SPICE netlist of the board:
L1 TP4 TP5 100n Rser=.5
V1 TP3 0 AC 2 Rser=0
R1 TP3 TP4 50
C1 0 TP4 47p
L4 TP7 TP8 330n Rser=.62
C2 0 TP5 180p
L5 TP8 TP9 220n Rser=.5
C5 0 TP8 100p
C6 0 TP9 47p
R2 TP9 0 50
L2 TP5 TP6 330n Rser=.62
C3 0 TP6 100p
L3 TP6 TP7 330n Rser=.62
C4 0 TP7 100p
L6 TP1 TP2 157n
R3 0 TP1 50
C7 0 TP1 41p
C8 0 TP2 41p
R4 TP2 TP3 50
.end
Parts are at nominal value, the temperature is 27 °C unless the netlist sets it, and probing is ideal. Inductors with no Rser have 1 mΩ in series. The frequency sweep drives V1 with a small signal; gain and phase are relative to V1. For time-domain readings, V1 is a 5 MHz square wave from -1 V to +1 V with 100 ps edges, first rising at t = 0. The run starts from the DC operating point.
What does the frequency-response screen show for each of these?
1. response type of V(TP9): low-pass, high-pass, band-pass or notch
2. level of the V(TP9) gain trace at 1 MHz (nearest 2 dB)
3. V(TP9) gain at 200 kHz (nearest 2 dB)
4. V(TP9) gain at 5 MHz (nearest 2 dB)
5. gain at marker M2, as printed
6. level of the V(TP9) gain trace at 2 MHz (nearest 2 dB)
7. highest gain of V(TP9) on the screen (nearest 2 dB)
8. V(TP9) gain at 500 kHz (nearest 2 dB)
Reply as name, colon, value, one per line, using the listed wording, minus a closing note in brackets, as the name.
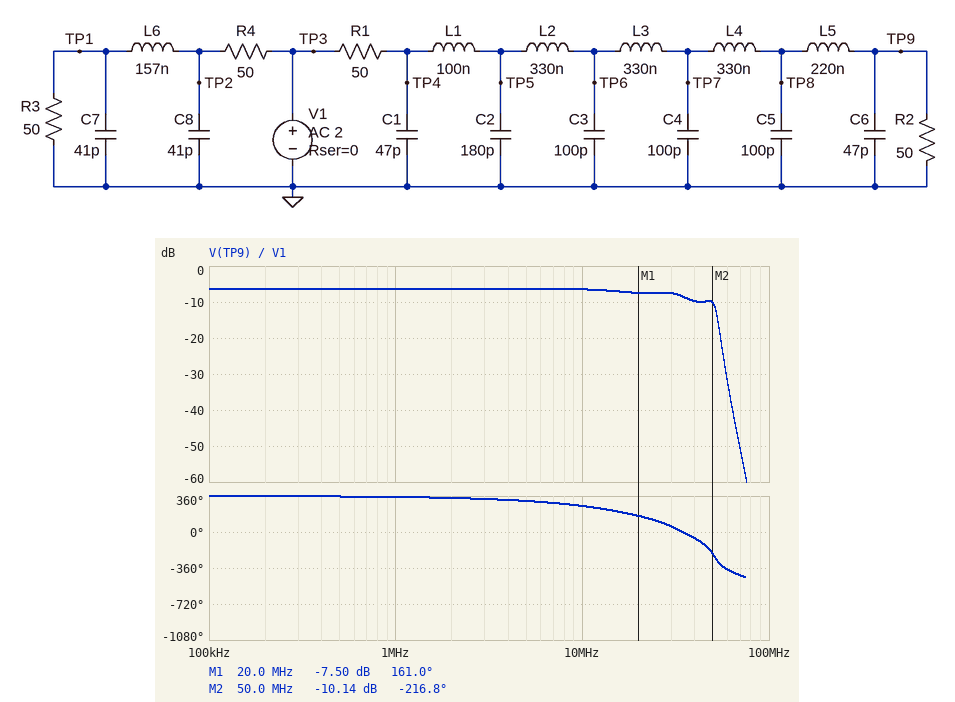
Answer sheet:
response type of V(TP9): low-pass, high-pass, band-pass or notch: low-pass
level of the V(TP9) gain trace at 1 MHz: -6 dB
V(TP9) gain at 200 kHz: -6 dB
V(TP9) gain at 5 MHz: -6 dB
gain at marker M2, as printed: -10.14 dB
level of the V(TP9) gain trace at 2 MHz: -6 dB
highest gain of V(TP9) on the screen: -6 dB
V(TP9) gain at 500 kHz: -6 dB
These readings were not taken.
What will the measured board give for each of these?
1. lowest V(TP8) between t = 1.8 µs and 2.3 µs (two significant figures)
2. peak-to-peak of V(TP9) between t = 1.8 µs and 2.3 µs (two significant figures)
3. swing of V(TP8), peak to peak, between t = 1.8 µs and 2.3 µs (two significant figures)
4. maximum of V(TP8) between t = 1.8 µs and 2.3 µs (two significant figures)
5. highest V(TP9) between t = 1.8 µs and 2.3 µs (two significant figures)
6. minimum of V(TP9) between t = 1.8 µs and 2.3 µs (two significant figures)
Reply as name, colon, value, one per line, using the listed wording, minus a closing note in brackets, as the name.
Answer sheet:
lowest V(TP8) between t = 1.8 µs and 2.3 µs: -590 mV
peak-to-peak of V(TP9) between t = 1.8 µs and 2.3 µs: 1.2 V
swing of V(TP8), peak to peak, between t = 1.8 µs and 2.3 µs: 1.2 V
maximum of V(TP8) between t = 1.8 µs and 2.3 µs: 590 mV
highest V(TP9) between t = 1.8 µs and 2.3 µs: 580 mV
minimum of V(TP9) between t = 1.8 µs and 2.3 µs: -580 mV
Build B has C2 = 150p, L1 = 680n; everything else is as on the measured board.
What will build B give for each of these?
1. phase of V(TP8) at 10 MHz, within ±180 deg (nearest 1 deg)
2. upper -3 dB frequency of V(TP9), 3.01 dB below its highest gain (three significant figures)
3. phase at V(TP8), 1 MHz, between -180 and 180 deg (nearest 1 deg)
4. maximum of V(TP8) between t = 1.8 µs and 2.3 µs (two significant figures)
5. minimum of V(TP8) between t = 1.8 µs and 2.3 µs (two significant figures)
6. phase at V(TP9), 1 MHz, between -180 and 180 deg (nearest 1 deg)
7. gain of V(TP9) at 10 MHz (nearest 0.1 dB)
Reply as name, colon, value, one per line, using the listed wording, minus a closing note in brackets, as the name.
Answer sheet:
phase of V(TP8) at 10 MHz, within ±180 deg: -100 deg
upper -3 dB frequency of V(TP9), 3.01 dB below its highest gain: 26.2 MHz
phase at V(TP8), 1 MHz, between -180 and 180 deg: -10 deg
maximum of V(TP8) between t = 1.8 µs and 2.3 µs: 570 mV
minimum of V(TP8) between t = 1.8 µs and 2.3 µs: -570 mV
phase at V(TP9), 1 MHz, between -180 and 180 deg: -12 deg
gain of V(TP9) at 10 MHz: -6.4 dB
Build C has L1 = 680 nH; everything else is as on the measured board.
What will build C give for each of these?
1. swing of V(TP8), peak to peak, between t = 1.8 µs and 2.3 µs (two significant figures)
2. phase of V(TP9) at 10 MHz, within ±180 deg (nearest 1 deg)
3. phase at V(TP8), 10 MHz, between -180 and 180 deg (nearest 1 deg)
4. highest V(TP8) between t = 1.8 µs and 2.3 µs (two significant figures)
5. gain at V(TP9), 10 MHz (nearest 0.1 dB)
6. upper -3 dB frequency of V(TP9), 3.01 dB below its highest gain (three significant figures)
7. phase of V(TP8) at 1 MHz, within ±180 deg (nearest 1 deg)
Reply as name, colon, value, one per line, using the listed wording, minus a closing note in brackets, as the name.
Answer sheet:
swing of V(TP8), peak to peak, between t = 1.8 µs and 2.3 µs: 1.1 V
phase of V(TP9) at 10 MHz, within ±180 deg: -120 deg
phase at V(TP8), 10 MHz, between -180 and 180 deg: -104 deg
highest V(TP8) between t = 1.8 µs and 2.3 µs: 560 mV
gain at V(TP9), 10 MHz: -6.3 dB
upper -3 dB frequency of V(TP9), 3.01 dB below its highest gain: 23.7 MHz
phase of V(TP8) at 1 MHz, within ±180 deg: -10 deg
